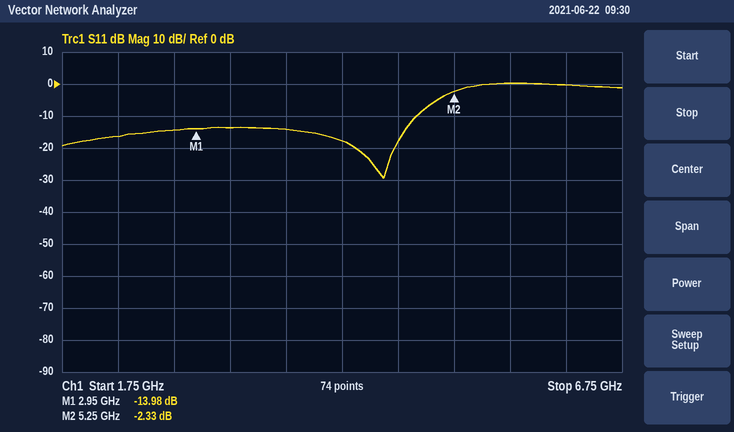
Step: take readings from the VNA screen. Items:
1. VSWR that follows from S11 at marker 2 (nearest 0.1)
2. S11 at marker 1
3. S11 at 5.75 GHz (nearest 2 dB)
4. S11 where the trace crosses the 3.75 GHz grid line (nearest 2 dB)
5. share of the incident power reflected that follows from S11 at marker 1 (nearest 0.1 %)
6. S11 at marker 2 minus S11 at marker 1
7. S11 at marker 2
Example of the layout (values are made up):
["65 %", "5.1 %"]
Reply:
["7.5", "-13.98 dB", "0 dB", "-14 dB", "4.0 %", "11.65 dB", "-2.33 dB"]
